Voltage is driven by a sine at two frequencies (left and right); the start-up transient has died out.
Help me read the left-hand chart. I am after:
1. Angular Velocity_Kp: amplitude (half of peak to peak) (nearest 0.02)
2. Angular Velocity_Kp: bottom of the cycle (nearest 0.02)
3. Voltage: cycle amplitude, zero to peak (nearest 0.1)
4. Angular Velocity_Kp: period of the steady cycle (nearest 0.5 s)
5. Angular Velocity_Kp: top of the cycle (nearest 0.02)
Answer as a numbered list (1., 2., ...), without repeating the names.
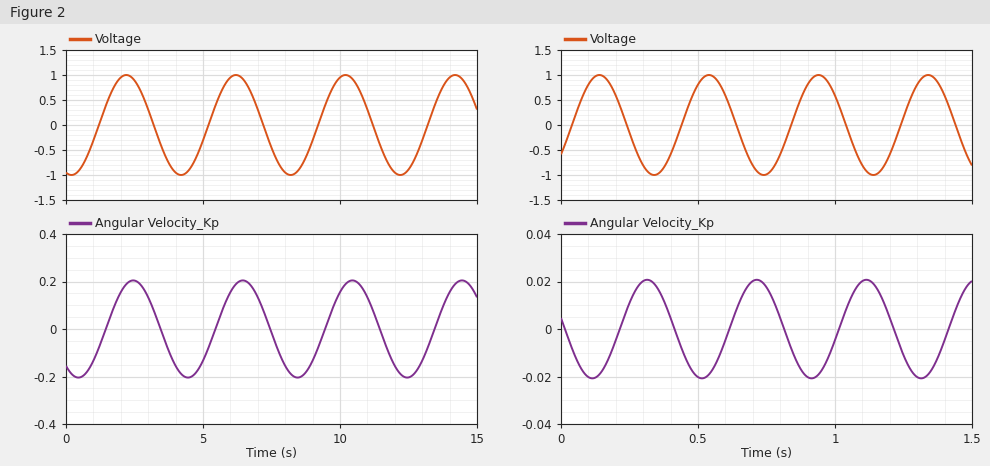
1. 0.20
2. -0.20
3. 1.0
4. 4.0 s
5. 0.20
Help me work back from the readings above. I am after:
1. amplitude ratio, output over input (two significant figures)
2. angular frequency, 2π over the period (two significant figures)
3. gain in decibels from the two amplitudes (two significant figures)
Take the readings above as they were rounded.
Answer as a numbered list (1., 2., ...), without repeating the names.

1. 0.20
2. 1.6 rad/s
3. -14 dB
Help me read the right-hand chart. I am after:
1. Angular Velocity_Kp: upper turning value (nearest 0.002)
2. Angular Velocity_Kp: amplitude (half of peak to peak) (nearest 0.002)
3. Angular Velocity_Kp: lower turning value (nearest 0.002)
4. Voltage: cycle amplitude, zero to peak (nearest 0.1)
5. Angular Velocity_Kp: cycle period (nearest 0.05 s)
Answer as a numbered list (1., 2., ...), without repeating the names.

1. 0.020
2. 0.020
3. -0.020
4. 1.0
5. 0.40 s
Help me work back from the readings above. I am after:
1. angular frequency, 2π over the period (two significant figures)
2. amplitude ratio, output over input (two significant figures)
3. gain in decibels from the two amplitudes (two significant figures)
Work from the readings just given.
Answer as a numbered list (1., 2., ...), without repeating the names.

1. 16 rad/s
2. 0.020
3. -34 dB
